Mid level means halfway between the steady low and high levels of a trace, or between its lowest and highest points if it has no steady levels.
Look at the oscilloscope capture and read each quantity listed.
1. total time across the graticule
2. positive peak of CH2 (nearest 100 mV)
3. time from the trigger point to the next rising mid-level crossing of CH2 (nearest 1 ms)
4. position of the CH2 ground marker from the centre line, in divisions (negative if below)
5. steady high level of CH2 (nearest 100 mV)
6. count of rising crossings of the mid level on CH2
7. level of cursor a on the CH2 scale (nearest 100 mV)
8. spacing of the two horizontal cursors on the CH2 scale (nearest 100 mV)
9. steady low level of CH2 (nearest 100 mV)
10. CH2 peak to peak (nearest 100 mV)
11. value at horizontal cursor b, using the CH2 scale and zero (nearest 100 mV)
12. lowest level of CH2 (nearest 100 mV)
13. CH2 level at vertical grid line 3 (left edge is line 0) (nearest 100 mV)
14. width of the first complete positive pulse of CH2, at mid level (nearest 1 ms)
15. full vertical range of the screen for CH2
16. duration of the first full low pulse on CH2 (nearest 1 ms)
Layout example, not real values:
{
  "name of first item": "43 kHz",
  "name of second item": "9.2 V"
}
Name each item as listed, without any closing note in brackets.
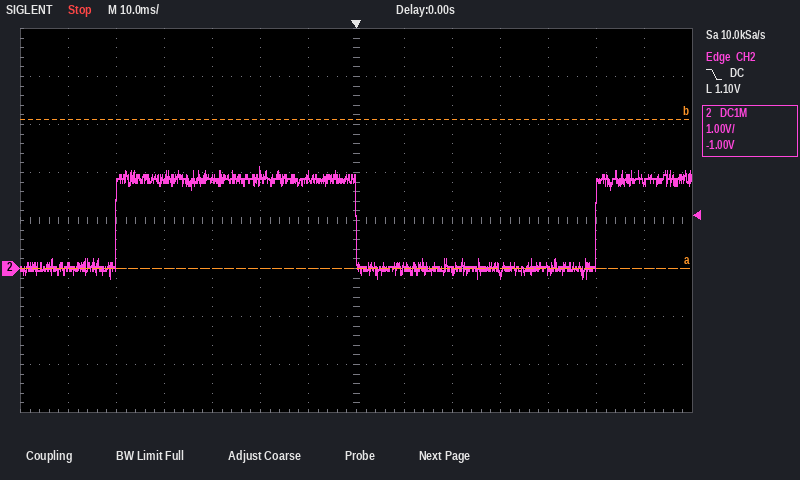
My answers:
{
  "total time across the graticule": "140 ms",
  "positive peak of CH2": "2.1 V",
  "time from the trigger point to the next rising mid-level crossing of CH2": "50 ms",
  "position of the CH2 ground marker from the centre line, in divisions": "-1.0 div",
  "steady high level of CH2": "1.9 V",
  "count of rising crossings of the mid level on CH2": "2",
  "level of cursor a on the CH2 scale": "0.0 V",
  "spacing of the two horizontal cursors on the CH2 scale": "3.1 V",
  "steady low level of CH2": "0.0 V",
  "CH2 peak to peak": "2.3 V",
  "value at horizontal cursor b, using the CH2 scale and zero": "3.1 V",
  "lowest level of CH2": "-200 mV",
  "CH2 level at vertical grid line 3 (left edge is line 0)": "1.9 V",
  "width of the first complete positive pulse of CH2, at mid level": "50 ms",
  "full vertical range of the screen for CH2": "8 V",
  "duration of the first full low pulse on CH2": "50 ms"
}
